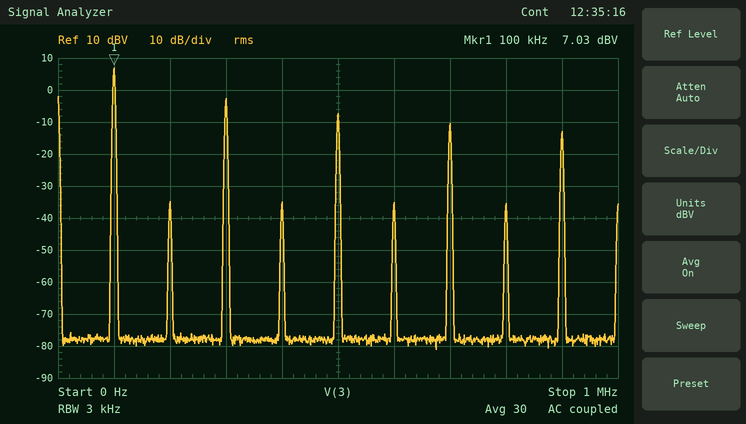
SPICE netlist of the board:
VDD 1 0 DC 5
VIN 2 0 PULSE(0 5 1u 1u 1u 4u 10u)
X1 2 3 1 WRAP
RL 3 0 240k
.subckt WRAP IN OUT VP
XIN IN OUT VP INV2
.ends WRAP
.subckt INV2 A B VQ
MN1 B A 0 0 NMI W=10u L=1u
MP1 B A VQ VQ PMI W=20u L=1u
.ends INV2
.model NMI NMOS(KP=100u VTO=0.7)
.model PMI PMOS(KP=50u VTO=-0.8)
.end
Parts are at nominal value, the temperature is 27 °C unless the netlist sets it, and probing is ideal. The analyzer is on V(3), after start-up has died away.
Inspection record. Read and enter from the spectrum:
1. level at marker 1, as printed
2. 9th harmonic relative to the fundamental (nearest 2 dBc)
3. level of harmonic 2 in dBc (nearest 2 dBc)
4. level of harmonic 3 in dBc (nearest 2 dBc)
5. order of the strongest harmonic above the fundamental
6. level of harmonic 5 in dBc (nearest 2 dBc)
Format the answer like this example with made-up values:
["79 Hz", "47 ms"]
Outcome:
["7.03 dBV", "-20 dBc", "-42 dBc", "-10 dBc", "3", "-14 dBc"]
